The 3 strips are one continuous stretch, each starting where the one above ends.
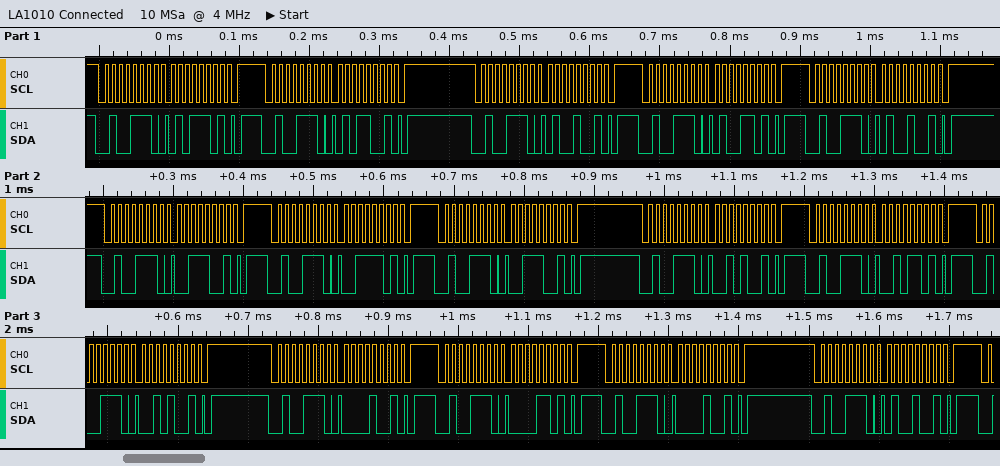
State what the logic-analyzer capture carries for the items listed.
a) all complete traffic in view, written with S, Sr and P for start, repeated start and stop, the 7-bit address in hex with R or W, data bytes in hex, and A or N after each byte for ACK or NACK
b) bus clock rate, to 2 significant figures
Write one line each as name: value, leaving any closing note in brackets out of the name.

all complete traffic in view, written with S, Sr and P for start, repeated start and stop, the 7-bit address in hex with R or W, data bytes in hex, and A or N after each byte for ACK or NACK: S 27W A 5D A P S 27W A 59 A P S 27W A 49 A P S 27W A 4D A P S 27W A 49 A P S 27W A 39 A P S 27W A 3D A P S 27W A 39 A P S 27W A 29 A P S 27W A 2D A P S 27W A 29 A P S 27W A 09 A P S 27W A 0D A P S 27W A 09 A P S 27W A 49 A P
bus clock rate, to 2 significant figures: 100 kHz
